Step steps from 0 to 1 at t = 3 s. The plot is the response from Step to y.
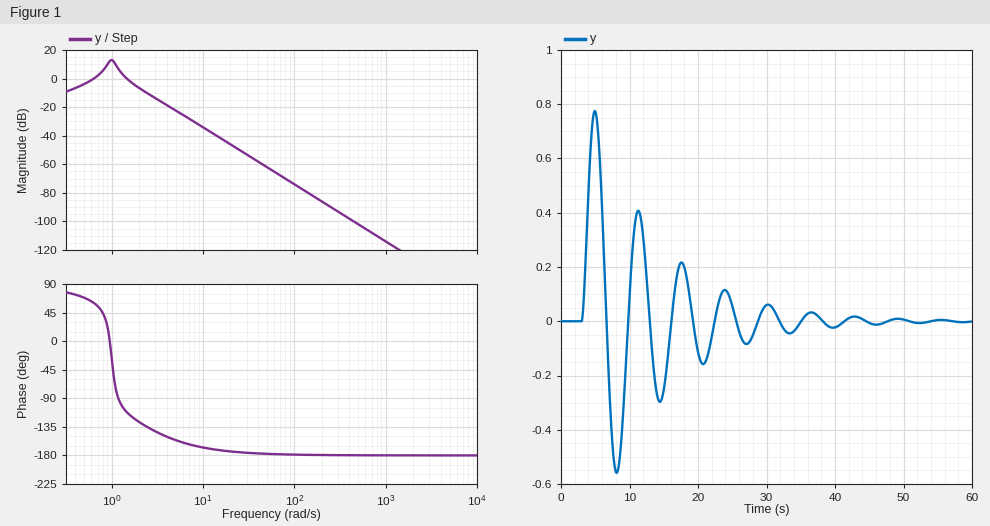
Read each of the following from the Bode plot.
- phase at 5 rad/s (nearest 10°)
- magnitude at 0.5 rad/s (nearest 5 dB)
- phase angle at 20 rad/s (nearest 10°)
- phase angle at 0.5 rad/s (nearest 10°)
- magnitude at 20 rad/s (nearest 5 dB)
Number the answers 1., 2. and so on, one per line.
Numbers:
1. -160°
2. -5 dB
3. -170°
4. 70°
5. -45 dB
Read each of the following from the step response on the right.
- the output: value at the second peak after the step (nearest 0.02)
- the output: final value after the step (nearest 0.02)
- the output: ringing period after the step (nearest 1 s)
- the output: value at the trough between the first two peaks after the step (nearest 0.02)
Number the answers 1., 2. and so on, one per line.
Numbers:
1. 0.40
2. 0.00
3. 6 s
4. -0.56
